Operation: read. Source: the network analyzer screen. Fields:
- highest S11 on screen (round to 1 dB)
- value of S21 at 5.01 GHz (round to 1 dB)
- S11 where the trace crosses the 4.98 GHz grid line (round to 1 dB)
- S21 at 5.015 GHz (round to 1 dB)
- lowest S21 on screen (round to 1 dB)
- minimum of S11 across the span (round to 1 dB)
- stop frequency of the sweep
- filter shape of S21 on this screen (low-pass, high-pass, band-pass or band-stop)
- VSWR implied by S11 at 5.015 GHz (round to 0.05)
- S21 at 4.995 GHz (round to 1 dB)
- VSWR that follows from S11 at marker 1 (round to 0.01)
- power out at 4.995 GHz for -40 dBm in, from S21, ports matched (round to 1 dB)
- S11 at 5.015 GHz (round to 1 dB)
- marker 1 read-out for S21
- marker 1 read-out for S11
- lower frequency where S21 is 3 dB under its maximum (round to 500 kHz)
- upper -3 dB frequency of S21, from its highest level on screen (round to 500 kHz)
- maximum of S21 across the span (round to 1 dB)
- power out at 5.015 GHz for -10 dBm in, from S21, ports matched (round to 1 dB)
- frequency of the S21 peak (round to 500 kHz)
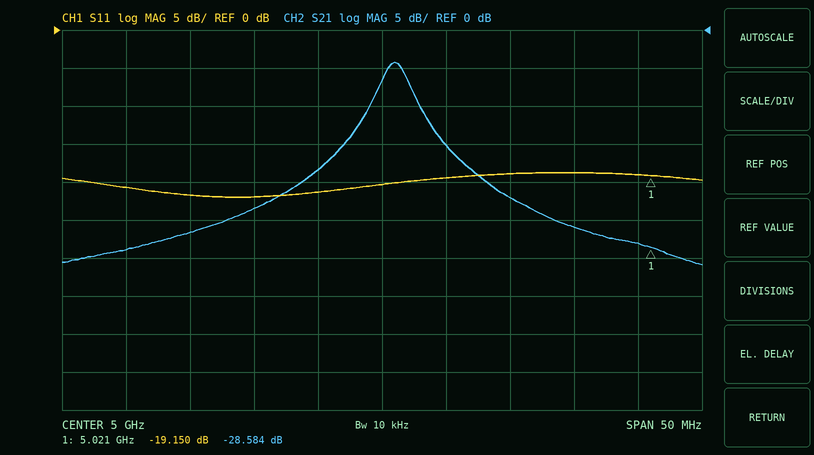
-19 dB
-22 dB
-21 dB
-26 dB
-31 dB
-22 dB
5.025 GHz
band-pass
1.25
-18 dB
1.25
-58 dBm
-19 dB
-28.584 dB
-19.150 dB
5.0000 GHz
5.0020 GHz
-4 dB
-36 dBm
5.0010 GHz
